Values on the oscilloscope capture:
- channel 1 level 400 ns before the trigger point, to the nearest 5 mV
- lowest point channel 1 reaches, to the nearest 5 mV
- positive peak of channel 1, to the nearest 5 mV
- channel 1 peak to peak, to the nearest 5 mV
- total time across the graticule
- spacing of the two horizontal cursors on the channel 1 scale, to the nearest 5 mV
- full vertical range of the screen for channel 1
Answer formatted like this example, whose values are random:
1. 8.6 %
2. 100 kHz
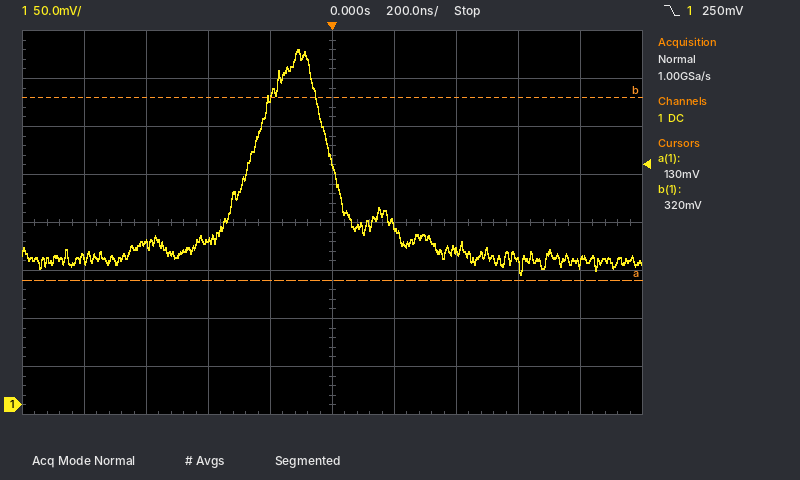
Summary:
1. 170 mV
2. 135 mV
3. 370 mV
4. 235 mV
5. 2 µs
6. 190 mV
7. 400 mV
